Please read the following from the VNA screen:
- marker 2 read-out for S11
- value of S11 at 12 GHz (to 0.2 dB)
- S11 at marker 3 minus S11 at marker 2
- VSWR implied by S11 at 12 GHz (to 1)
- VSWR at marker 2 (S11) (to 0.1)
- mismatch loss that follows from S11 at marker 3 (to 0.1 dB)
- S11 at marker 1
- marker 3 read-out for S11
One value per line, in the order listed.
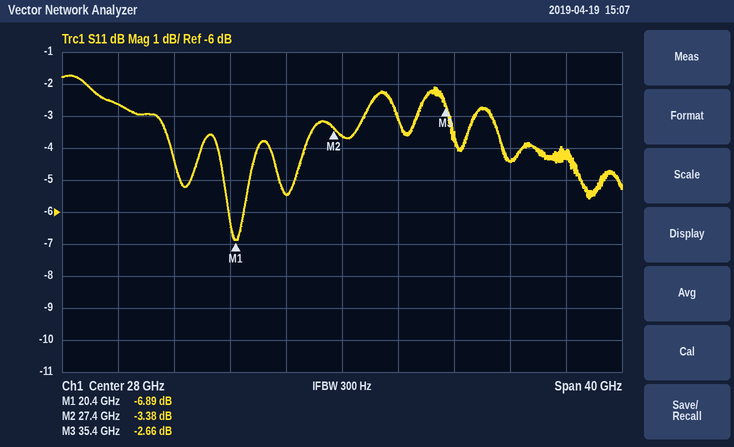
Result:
-3.38 dB
-2.6 dB
0.72 dB
7
5.2
3.4 dB
-6.89 dB
-2.66 dB
